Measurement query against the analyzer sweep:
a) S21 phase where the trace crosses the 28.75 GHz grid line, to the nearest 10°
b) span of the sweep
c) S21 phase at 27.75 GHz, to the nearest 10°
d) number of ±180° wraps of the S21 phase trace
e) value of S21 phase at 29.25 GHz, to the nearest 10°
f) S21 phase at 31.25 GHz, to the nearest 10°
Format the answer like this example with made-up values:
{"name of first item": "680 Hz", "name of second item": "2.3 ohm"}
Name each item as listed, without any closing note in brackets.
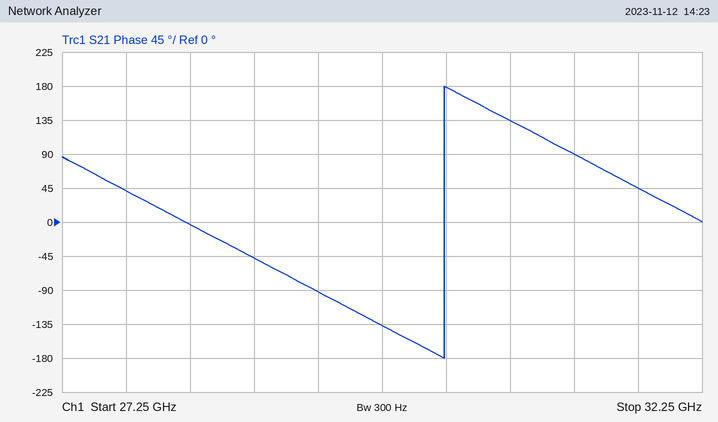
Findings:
{"S21 phase where the trace crosses the 28.75 GHz grid line, to the nearest 10°": "-50°", "span of the sweep": "5 GHz", "S21 phase at 27.75 GHz, to the nearest 10°": "40°", "number of ±180° wraps of the S21 phase trace": "1", "value of S21 phase at 29.25 GHz, to the nearest 10°": "-90°", "S21 phase at 31.25 GHz, to the nearest 10°": "90°"}
